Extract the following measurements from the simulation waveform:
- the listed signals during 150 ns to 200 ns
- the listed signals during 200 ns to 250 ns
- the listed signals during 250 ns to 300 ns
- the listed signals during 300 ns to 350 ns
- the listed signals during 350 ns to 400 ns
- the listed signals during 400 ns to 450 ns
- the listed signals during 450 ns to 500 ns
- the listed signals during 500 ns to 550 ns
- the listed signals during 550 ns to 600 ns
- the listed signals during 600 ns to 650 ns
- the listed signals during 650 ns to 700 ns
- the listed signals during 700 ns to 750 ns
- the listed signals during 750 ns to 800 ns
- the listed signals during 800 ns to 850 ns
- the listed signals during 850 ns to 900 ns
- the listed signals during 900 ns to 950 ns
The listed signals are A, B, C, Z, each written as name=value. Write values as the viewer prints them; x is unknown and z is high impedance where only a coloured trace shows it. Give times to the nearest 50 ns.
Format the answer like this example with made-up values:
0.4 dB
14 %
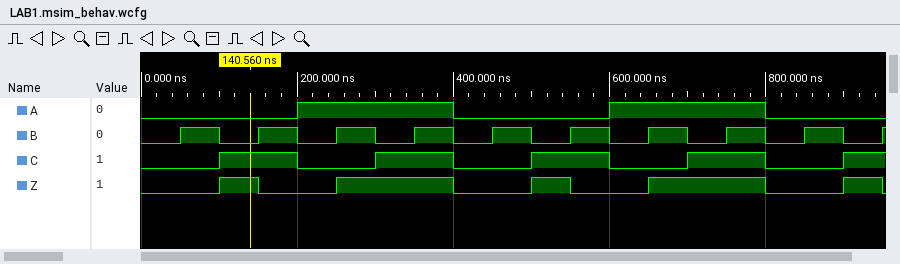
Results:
A=0, B=1, C=1, Z=0
A=1, B=0, C=0, Z=0
A=1, B=1, C=0, Z=1
A=1, B=0, C=1, Z=1
A=1, B=1, C=1, Z=1
A=0, B=0, C=0, Z=0
A=0, B=1, C=0, Z=0
A=0, B=0, C=1, Z=1
A=0, B=1, C=1, Z=0
A=1, B=0, C=0, Z=0
A=1, B=1, C=0, Z=1
A=1, B=0, C=1, Z=1
A=1, B=1, C=1, Z=1
A=0, B=0, C=0, Z=0
A=0, B=1, C=0, Z=0
A=0, B=0, C=1, Z=1
